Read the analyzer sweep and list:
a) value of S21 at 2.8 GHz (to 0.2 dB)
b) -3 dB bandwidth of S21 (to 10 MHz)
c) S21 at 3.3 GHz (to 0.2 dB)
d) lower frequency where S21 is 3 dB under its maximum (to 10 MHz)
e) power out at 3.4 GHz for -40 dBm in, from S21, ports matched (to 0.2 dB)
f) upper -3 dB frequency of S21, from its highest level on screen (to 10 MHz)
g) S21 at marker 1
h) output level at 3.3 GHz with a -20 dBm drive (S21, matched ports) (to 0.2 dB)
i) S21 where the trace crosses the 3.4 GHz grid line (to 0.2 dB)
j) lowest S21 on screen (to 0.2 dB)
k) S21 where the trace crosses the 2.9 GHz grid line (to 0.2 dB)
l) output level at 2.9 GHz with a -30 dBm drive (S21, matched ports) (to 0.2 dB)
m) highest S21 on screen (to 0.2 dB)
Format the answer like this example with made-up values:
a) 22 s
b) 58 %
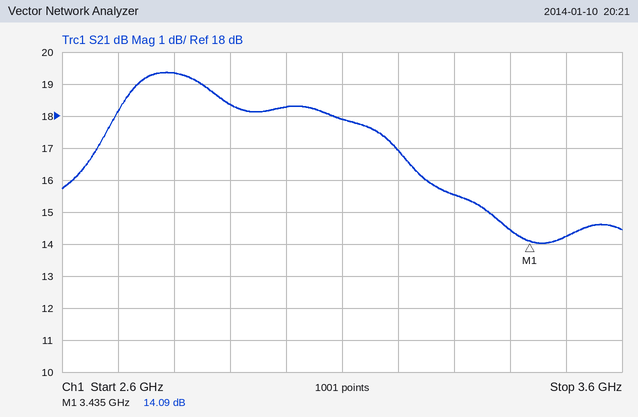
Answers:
a) 19.4 dB
b) 590 MHz
c) 15.6 dB
d) 2.64 GHz
e) -25.6 dBm
f) 3.23 GHz
g) 14.09 dB
h) -4.4 dBm
i) 14.4 dB
j) 14.0 dB
k) 18.4 dB
l) -11.6 dBm
m) 19.4 dB
